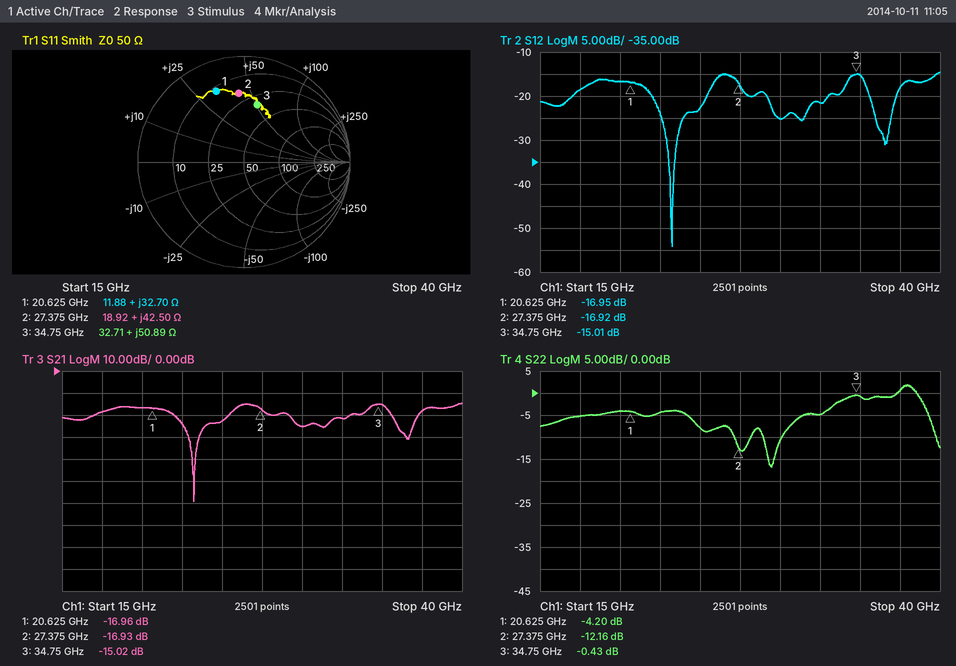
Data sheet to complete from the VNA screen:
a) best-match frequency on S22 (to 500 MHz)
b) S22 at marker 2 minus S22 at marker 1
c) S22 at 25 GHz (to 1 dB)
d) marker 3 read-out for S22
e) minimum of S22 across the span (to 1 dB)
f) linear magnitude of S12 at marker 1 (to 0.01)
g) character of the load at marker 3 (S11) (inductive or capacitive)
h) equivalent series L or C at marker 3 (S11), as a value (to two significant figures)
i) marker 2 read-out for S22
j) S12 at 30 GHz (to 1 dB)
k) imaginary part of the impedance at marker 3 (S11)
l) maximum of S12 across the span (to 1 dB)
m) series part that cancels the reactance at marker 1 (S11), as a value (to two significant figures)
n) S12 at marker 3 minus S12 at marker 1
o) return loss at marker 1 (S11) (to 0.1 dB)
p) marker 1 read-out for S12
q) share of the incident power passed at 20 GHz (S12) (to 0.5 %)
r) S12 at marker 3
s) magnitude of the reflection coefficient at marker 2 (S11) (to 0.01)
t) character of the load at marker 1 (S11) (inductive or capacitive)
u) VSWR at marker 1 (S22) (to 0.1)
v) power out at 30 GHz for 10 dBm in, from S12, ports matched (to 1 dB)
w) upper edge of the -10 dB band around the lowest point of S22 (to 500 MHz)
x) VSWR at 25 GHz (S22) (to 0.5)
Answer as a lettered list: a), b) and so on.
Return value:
a) 29.5 GHz
b) -7.96 dB
c) -8 dB
d) -0.43 dB
e) -17 dB
f) 0.14
g) inductive
h) 230 pH
i) -12.16 dB
j) -25 dB
k) +50.89 Ω
l) -15 dB
m) 240 fF
n) 1.94 dB
o) 2.9 dB
p) -16.95 dB
q) 2.0 %
r) -15.01 dB
s) 0.65
t) inductive
u) 4.2
v) -15 dBm
w) 30.0 GHz
x) 2.5
